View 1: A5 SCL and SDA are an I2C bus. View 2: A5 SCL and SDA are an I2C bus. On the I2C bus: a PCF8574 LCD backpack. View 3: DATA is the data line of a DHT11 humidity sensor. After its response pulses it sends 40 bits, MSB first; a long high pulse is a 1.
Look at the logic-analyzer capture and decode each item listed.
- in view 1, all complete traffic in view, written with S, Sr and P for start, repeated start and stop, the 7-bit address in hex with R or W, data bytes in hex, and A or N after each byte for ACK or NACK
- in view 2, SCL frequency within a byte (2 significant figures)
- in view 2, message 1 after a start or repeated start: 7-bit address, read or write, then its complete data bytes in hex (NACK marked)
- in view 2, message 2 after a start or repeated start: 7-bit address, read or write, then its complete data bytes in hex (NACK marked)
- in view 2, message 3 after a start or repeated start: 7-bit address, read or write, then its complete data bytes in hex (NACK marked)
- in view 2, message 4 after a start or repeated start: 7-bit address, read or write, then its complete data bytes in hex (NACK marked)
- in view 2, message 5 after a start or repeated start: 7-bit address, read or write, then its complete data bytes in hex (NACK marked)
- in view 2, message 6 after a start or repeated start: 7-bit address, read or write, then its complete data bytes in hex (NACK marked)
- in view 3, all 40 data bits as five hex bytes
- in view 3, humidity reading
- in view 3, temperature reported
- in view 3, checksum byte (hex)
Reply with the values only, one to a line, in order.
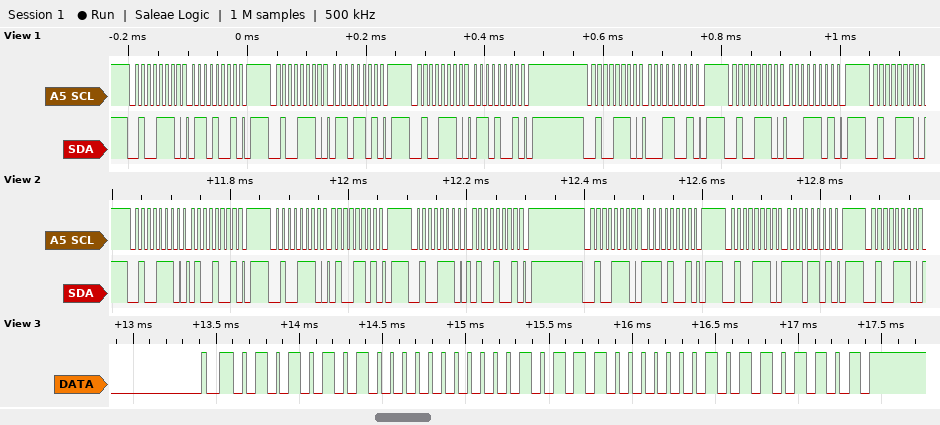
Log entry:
S 27W A 69 A P S 27W A 6D A P S 27W A 69 A P S 27W A 19 A P S 27W A 1D A P S 27W A
100 kHz
0x27 write: 49
0x27 write: 4D
0x27 write: 49
0x27 write: E9
0x27 write: ED
0x27 write
55 00 17 01 6D
85 %
23.1 °C
0x6D
